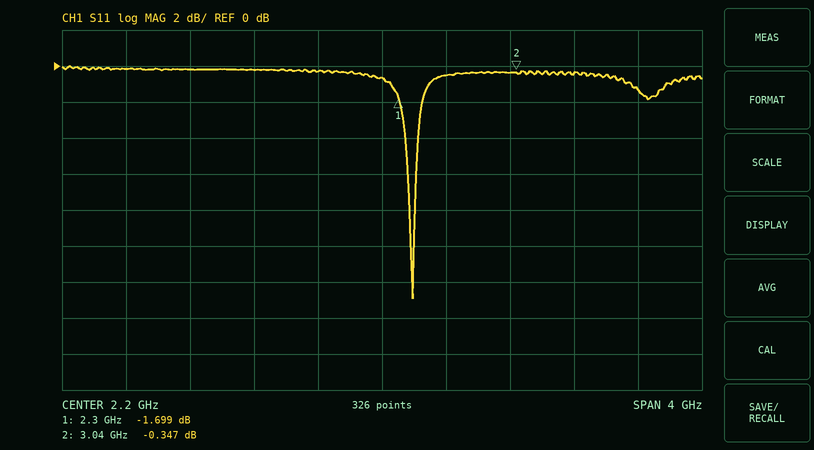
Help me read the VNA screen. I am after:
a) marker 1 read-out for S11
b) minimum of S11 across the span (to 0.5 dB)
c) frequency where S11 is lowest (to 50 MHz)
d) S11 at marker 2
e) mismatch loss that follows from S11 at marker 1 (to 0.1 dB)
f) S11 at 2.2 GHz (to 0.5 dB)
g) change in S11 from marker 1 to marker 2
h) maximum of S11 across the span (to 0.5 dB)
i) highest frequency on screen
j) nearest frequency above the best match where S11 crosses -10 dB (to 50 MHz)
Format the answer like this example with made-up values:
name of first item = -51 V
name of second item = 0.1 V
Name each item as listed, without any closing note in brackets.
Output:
marker 1 read-out for S11 = -1.699 dB
minimum of S11 across the span = -13.0 dB
frequency where S11 is lowest = 2.40 GHz
S11 at marker 2 = -0.347 dB
mismatch loss that follows from S11 at marker 1 = 4.9 dB
S11 at 2.2 GHz = -0.5 dB
change in S11 from marker 1 to marker 2 = 1.352 dB
maximum of S11 across the span = 0.0 dB
highest frequency on screen = 4.2 GHz
nearest frequency above the best match where S11 crosses -10 dB = 2.40 GHz
